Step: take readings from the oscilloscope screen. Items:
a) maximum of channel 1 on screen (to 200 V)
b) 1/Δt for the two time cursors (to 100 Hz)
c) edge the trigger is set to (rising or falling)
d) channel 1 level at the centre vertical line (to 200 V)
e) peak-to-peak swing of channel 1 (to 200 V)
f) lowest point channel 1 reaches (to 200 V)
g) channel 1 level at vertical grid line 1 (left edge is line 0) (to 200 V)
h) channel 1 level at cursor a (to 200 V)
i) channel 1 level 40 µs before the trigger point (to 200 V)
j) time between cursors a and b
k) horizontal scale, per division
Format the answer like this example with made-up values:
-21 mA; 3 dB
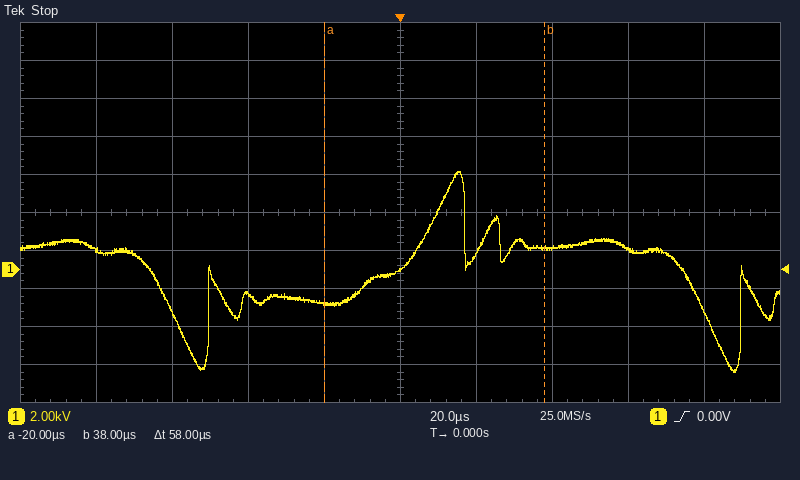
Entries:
5.2 kV; 17.2 kHz; rising; 0.0 kV; 10.6 kV; -5.4 kV; 1.0 kV; -1.8 kV; -1.4 kV; 58 µs; 20 µs
